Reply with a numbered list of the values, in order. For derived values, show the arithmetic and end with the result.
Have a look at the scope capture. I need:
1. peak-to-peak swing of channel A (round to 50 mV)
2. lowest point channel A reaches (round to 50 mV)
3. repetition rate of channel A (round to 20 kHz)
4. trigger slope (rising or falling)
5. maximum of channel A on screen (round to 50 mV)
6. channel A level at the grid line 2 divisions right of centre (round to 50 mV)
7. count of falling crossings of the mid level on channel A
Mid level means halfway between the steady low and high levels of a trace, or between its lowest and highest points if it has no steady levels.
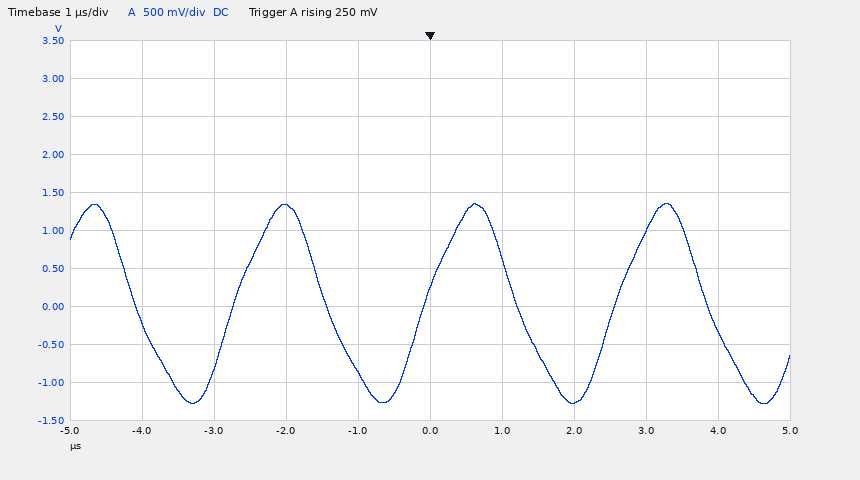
1. 1.35 V − (-1.30 V) = 2.65 V
2. -1.30 V
3. 380 kHz
4. rising
5. 1.35 V
6. -1.25 V
7. 4
